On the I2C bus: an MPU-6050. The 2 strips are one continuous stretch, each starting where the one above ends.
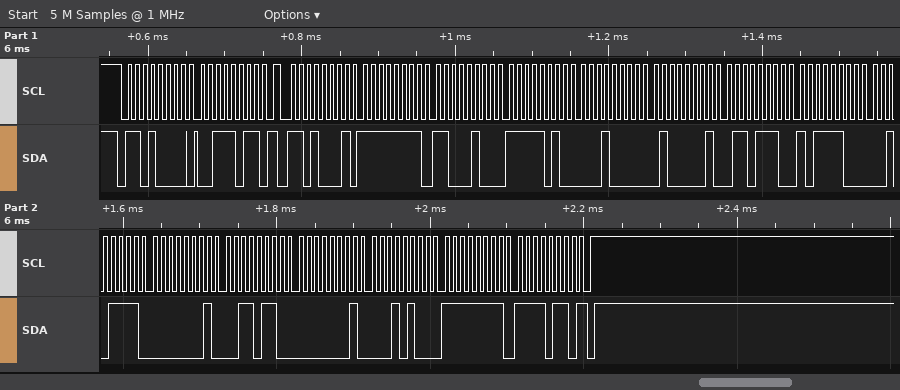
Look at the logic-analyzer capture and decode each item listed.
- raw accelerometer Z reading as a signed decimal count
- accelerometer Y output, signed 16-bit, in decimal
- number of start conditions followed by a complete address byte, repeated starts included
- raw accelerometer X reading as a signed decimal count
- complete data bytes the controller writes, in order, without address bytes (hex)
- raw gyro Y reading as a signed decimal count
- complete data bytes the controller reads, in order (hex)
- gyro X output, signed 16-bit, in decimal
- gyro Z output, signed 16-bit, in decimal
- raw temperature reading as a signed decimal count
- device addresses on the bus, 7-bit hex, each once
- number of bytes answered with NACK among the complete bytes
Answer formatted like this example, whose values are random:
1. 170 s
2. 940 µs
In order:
1. 16750
2. -1520
3. 2
4. -60
5. 3B
6. 276
7. FF C4 FA 10 41 6E BC 2F 01 36 01 14 FF F6
8. 310
9. -10
10. -17361
11. 0x68
12. 1
